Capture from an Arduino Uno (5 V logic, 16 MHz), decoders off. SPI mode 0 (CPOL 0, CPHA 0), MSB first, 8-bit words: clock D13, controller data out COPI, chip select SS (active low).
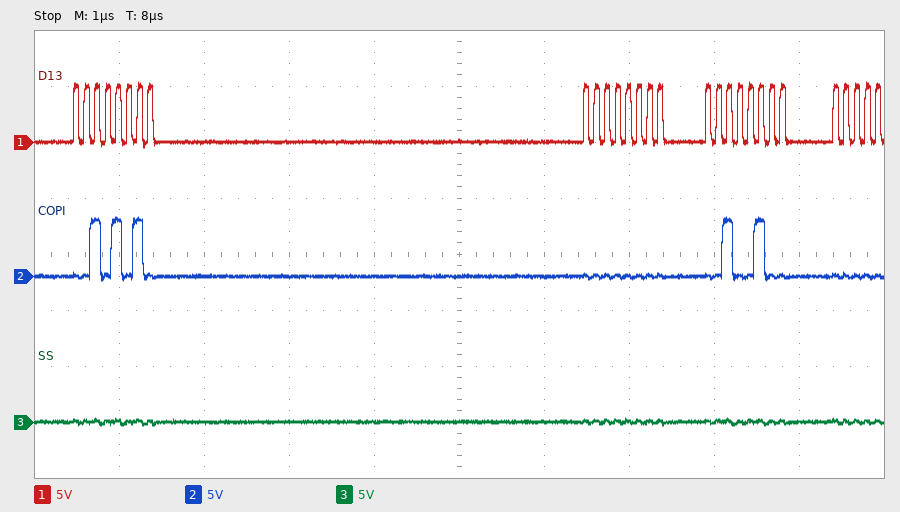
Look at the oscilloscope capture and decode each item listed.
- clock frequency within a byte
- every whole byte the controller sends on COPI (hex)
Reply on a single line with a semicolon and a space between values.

8 MHz; 2A 00 24
